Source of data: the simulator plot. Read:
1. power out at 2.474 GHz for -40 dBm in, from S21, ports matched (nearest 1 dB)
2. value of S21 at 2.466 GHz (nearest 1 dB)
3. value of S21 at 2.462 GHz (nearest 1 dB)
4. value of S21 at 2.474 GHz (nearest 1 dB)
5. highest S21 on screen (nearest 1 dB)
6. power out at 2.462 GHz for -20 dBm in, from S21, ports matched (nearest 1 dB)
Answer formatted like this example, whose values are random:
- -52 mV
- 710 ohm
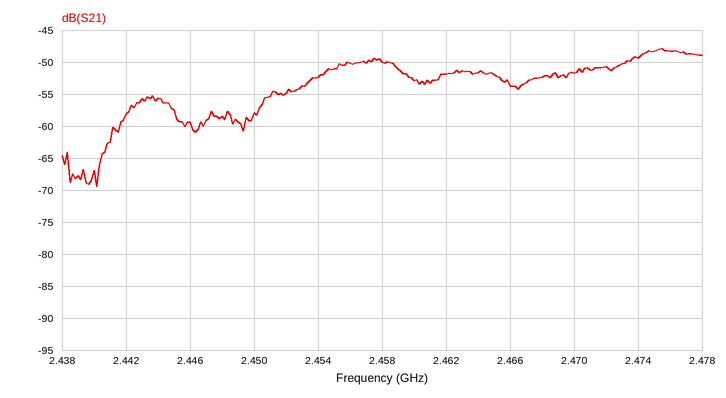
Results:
- -89 dBm
- -54 dB
- -52 dB
- -49 dB
- -48 dB
- -72 dBm
